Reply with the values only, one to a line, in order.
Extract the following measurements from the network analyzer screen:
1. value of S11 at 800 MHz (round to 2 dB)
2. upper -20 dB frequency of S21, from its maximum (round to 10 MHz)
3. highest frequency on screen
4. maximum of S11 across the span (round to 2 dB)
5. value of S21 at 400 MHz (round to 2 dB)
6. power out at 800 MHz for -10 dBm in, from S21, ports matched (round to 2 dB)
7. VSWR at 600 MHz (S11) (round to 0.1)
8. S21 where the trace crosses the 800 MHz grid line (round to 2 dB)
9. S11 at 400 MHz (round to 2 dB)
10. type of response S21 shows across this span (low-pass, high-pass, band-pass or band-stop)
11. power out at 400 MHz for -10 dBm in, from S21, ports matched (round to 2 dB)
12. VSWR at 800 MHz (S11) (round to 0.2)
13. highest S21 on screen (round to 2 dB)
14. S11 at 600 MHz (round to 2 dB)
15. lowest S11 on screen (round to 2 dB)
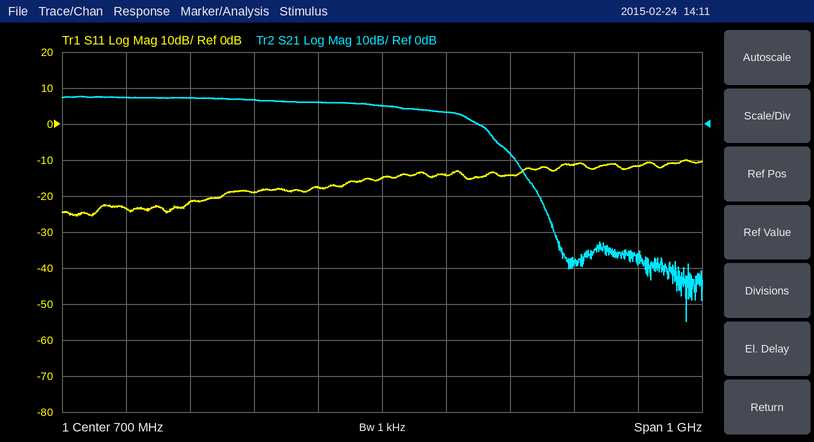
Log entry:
-14 dB
920 MHz
1.2 GHz
-10 dB
8 dB
-6 dBm
1.3
4 dB
-22 dB
low-pass
-2 dBm
1.4
8 dB
-18 dB
-26 dB
